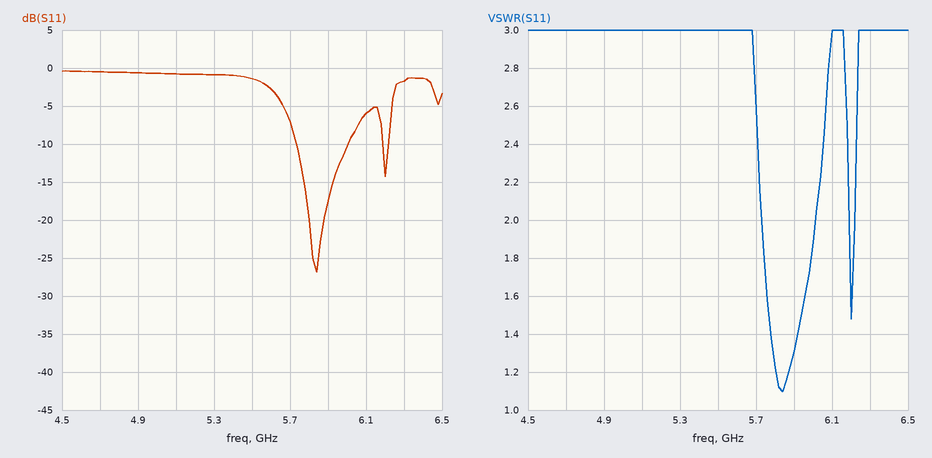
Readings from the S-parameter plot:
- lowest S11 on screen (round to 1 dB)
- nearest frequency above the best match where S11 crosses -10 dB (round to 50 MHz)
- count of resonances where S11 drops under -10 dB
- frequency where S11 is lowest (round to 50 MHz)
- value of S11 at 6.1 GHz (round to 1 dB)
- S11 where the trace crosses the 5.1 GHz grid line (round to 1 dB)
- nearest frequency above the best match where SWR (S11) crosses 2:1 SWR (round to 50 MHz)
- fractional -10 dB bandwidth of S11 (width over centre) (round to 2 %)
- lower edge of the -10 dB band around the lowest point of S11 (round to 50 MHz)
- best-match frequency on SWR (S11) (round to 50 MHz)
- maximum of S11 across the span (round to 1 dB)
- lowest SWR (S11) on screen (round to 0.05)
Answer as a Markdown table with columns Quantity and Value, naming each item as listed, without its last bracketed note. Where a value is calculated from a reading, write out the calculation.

| Quantity | Value |
|---|---|
| lowest S11 on screen | -27 dB |
| nearest frequency above the best match where S11 crosses -10 dB | 6.00 GHz |
| count of resonances where S11 drops under -10 dB | 2 |
| frequency where S11 is lowest | 5.85 GHz |
| value of S11 at 6.1 GHz | -6 dB |
| S11 where the trace crosses the 5.1 GHz grid line | -1 dB |
| nearest frequency above the best match where SWR (S11) crosses 2:1 SWR | 6.00 GHz |
| fractional -10 dB bandwidth of S11 (width over centre) | 250 MHz / 5.875 GHz ≈ 4 % |
| lower edge of the -10 dB band around the lowest point of S11 | 5.75 GHz |
| best-match frequency on SWR (S11) | 5.85 GHz |
| maximum of S11 across the span | 0 dB |
| lowest SWR (S11) on screen | 1.10 |
